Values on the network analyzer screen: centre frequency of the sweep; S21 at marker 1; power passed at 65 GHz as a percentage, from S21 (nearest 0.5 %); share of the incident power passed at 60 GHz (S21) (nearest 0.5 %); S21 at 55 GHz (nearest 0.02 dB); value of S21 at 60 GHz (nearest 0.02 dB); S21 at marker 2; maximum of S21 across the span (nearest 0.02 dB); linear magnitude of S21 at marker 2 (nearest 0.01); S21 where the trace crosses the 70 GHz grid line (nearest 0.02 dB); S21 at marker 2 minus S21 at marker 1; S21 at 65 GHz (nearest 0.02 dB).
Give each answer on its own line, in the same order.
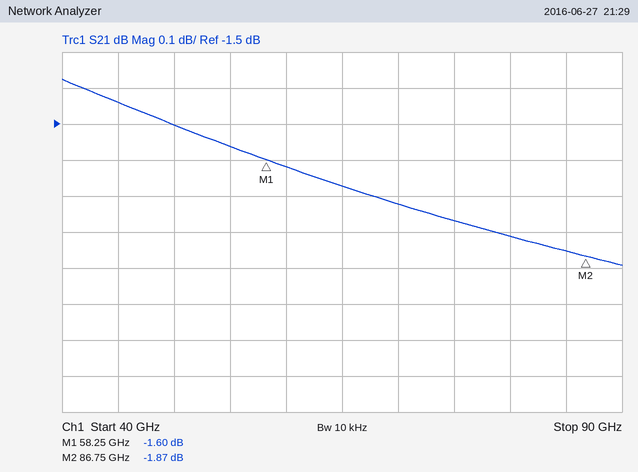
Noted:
65 GHz
-1.60 dB
68.0 %
69.0 %
-1.56 dB
-1.62 dB
-1.87 dB
-1.38 dB
0.81
-1.72 dB
-0.27 dB
-1.68 dB
